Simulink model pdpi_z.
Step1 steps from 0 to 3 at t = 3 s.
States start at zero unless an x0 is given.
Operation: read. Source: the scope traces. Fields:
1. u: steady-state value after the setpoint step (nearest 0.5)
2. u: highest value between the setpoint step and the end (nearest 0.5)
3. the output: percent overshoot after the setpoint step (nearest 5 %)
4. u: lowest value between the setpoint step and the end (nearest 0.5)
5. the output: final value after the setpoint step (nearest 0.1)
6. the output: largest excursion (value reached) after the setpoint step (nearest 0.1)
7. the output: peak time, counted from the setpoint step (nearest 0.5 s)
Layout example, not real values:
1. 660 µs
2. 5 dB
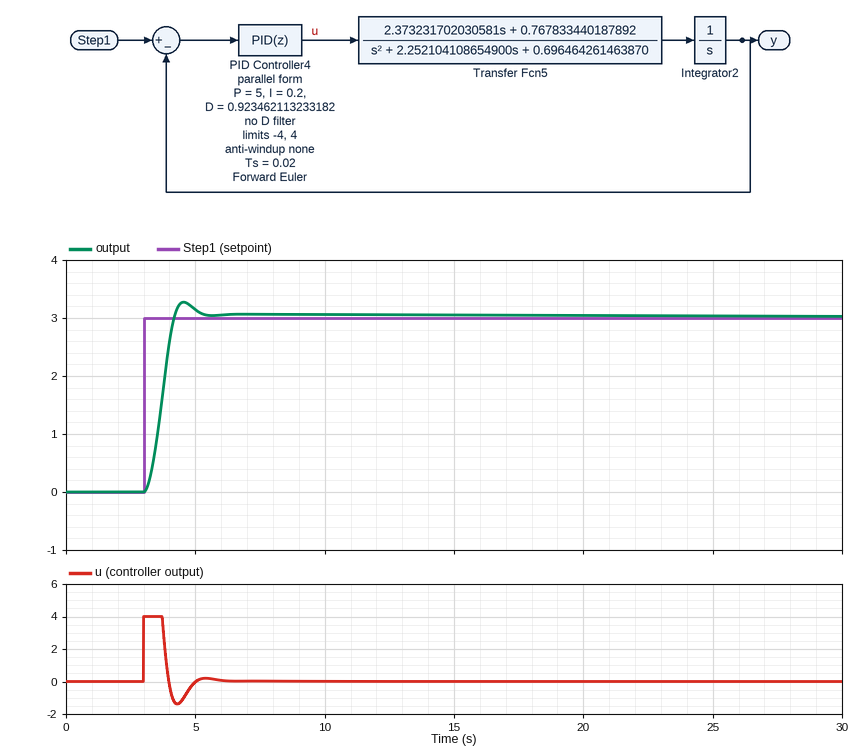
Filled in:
1. 0.0
2. 4.0
3. 10 %
4. -1.5
5. 3.0
6. 3.3
7. 1.5 s
